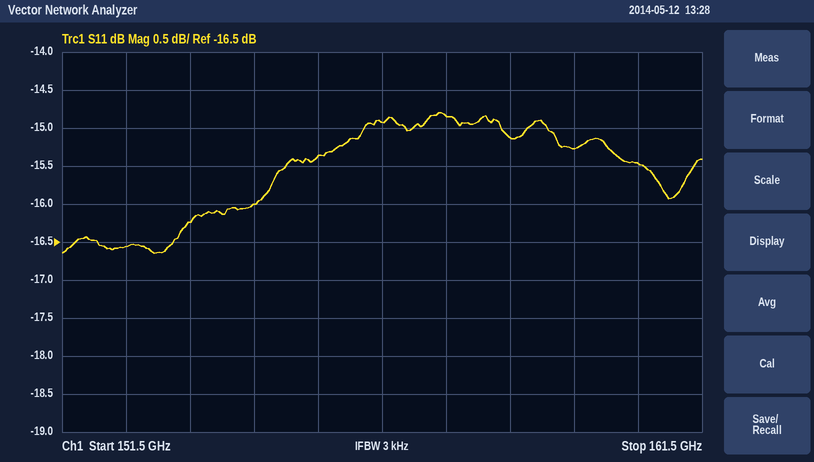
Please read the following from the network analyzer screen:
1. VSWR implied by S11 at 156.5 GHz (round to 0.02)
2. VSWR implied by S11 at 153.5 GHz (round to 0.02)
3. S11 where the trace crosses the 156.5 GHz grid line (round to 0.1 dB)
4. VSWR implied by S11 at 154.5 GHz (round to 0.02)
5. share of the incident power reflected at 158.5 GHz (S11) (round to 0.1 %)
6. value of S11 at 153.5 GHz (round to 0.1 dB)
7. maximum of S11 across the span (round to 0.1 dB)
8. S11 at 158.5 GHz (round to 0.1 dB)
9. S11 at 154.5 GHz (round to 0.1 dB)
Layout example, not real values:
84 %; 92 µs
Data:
1.44; 1.36; -14.9 dB; 1.38; 3.1 %; -16.2 dB; -14.8 dB; -15.1 dB; -16.0 dB
